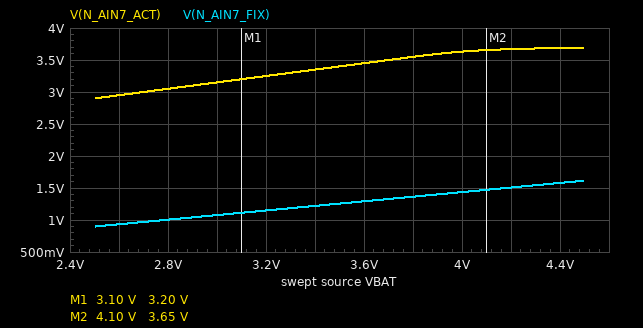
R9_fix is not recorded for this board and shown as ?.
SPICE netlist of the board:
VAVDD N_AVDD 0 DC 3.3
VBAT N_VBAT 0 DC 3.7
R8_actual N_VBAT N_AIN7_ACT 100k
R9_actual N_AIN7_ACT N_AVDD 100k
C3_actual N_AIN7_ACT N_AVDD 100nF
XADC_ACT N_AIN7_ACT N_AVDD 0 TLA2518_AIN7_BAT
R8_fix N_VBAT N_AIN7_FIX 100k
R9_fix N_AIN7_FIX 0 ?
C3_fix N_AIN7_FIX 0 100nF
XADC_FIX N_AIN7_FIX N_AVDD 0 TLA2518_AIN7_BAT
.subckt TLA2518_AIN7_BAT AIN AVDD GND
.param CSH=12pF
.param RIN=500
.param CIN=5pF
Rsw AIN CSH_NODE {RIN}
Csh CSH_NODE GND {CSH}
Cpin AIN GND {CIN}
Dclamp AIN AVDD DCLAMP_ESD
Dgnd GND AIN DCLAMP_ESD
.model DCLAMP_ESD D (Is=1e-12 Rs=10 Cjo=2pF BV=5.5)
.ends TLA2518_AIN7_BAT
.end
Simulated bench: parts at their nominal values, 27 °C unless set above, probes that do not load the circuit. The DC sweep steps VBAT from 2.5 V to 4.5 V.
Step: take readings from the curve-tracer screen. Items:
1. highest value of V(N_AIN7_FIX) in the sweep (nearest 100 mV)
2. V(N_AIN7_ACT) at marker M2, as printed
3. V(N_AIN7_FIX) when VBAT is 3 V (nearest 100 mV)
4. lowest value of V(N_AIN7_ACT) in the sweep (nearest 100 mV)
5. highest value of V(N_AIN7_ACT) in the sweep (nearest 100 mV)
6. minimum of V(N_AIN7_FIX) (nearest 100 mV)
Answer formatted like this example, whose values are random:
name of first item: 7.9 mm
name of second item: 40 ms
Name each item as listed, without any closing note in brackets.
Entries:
highest value of V(N_AIN7_FIX) in the sweep: 1.6 V
V(N_AIN7_ACT) at marker M2, as printed: 3.65 V
V(N_AIN7_FIX) when VBAT is 3 V: 1.1 V
lowest value of V(N_AIN7_ACT) in the sweep: 2.9 V
highest value of V(N_AIN7_ACT) in the sweep: 3.7 V
minimum of V(N_AIN7_FIX): 900 mV
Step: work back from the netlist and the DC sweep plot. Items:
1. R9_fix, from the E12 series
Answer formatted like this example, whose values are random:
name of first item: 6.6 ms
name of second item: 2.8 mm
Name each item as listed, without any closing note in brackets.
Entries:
R9_fix, from the E12 series: 56 kΩ
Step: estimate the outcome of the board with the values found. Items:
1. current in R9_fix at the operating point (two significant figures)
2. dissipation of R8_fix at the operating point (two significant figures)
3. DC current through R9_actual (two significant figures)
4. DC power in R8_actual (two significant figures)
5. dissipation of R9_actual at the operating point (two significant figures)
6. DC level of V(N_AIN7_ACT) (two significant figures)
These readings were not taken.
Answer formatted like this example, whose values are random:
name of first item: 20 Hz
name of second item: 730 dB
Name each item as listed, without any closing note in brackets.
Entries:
current in R9_fix at the operating point: 24 µA
dissipation of R8_fix at the operating point: 56 µW
DC current through R9_actual: 2.0 µA
DC power in R8_actual: 400 nW
dissipation of R9_actual at the operating point: 400 nW
DC level of V(N_AIN7_ACT): 3.5 V
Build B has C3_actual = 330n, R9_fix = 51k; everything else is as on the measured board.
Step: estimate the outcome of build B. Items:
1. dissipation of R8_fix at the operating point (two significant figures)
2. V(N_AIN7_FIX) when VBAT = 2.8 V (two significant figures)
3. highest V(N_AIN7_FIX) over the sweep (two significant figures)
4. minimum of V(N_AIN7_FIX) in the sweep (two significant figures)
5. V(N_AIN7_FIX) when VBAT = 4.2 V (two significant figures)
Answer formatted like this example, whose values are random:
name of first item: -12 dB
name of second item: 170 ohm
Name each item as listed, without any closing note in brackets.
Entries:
dissipation of R8_fix at the operating point: 60 µW
V(N_AIN7_FIX) when VBAT = 2.8 V: 950 mV
highest V(N_AIN7_FIX) over the sweep: 1.5 V
minimum of V(N_AIN7_FIX) in the sweep: 840 mV
V(N_AIN7_FIX) when VBAT = 4.2 V: 1.4 V
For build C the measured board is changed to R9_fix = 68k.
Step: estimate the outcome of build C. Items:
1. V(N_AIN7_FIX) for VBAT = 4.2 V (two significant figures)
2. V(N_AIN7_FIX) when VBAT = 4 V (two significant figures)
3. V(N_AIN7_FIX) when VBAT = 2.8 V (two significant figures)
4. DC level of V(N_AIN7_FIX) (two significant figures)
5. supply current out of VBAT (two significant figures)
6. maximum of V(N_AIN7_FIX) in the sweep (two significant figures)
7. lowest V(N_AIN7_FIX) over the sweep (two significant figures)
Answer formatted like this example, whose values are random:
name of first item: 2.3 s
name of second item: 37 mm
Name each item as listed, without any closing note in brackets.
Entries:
V(N_AIN7_FIX) for VBAT = 4.2 V: 1.7 V
V(N_AIN7_FIX) when VBAT = 4 V: 1.6 V
V(N_AIN7_FIX) when VBAT = 2.8 V: 1.1 V
DC level of V(N_AIN7_FIX): 1.5 V
supply current out of VBAT: 24 µA
maximum of V(N_AIN7_FIX) in the sweep: 1.8 V
lowest V(N_AIN7_FIX) over the sweep: 1.0 V
